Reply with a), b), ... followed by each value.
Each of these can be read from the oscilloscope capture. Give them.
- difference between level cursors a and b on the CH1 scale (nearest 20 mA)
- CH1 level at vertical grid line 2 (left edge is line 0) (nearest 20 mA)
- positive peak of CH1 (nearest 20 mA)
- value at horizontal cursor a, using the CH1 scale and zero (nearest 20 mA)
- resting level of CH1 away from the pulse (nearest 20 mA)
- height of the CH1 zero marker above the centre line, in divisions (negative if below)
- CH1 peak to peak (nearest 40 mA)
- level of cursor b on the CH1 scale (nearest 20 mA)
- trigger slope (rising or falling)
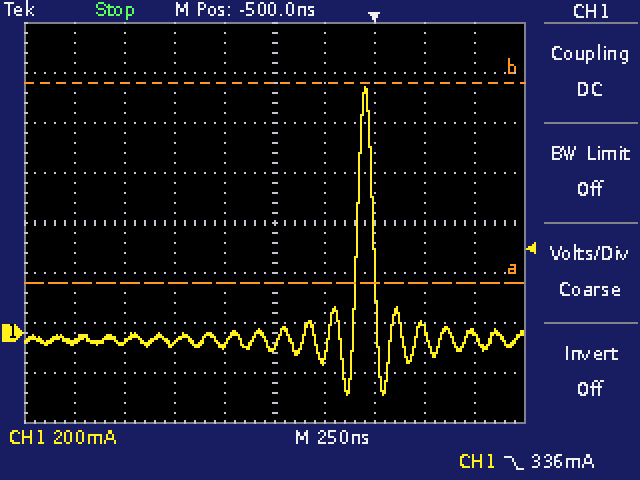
a) 800 mA
b) -40 mA
c) 980 mA
d) 200 mA
e) -20 mA
f) -2.2 div
g) 1.24 A
h) 1.00 A
i) falling
